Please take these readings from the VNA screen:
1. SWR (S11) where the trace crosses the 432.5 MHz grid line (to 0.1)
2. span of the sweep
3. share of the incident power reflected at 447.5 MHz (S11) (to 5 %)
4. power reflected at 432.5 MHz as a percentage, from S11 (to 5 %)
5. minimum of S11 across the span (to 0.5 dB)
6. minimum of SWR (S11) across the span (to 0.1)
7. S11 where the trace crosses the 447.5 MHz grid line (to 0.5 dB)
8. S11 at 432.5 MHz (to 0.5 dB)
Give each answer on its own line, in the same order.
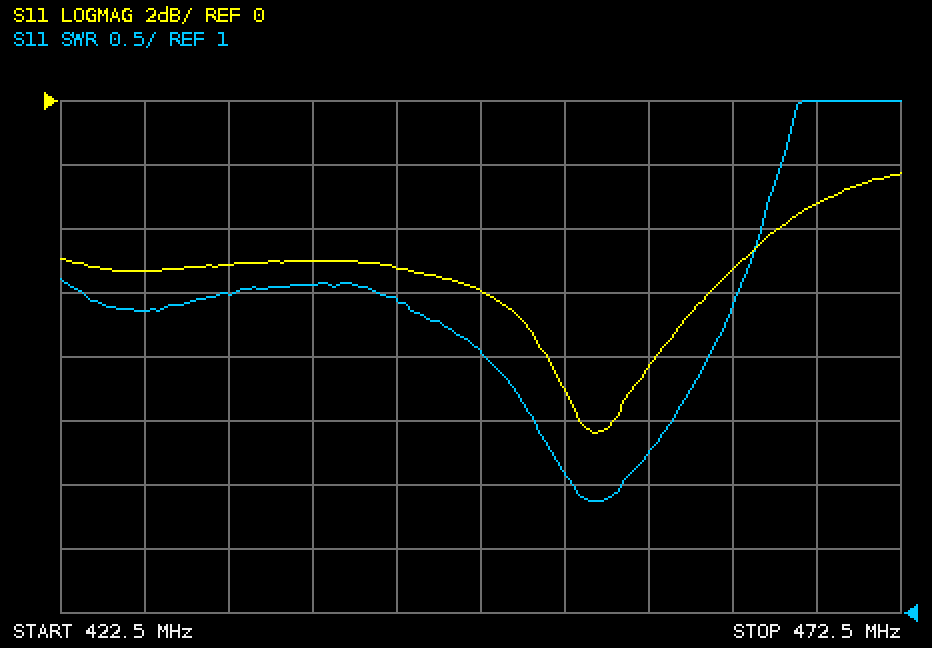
3.5
50 MHz
25 %
30 %
-10.5 dB
1.9
-6.0 dB
-5.0 dB
